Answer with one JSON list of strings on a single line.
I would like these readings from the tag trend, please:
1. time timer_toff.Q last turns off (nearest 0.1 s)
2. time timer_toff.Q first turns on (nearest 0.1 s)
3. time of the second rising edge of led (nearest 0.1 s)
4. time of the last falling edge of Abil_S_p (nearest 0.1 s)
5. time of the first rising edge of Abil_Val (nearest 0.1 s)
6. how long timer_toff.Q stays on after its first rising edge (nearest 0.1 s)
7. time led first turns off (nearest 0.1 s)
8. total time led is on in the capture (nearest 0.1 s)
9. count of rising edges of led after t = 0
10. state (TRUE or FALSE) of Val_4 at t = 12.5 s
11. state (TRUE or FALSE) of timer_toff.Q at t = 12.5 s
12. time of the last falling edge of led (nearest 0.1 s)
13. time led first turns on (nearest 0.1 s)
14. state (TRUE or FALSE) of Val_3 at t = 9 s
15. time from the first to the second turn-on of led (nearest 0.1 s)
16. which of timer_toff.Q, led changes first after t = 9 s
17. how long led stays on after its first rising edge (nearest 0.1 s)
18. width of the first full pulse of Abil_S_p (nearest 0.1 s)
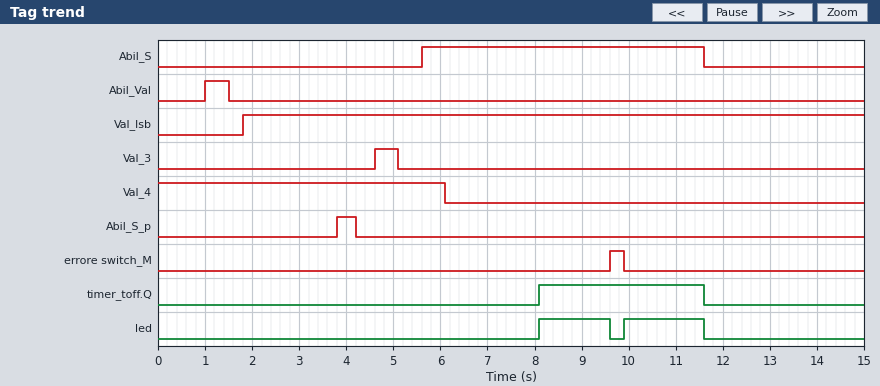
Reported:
["11.6 s", "8.1 s", "9.9 s", "4.2 s", "1.0 s", "3.5 s", "9.6 s", "3.2 s", "2", "FALSE", "FALSE", "11.6 s", "8.1 s", "FALSE", "1.8 s", "led", "1.5 s", "0.4 s"]
